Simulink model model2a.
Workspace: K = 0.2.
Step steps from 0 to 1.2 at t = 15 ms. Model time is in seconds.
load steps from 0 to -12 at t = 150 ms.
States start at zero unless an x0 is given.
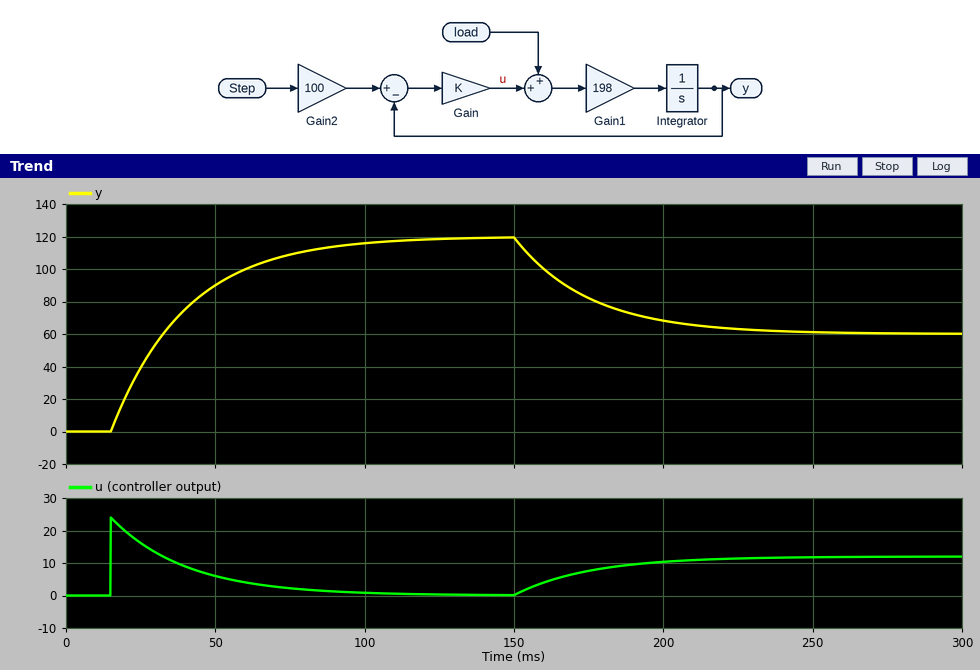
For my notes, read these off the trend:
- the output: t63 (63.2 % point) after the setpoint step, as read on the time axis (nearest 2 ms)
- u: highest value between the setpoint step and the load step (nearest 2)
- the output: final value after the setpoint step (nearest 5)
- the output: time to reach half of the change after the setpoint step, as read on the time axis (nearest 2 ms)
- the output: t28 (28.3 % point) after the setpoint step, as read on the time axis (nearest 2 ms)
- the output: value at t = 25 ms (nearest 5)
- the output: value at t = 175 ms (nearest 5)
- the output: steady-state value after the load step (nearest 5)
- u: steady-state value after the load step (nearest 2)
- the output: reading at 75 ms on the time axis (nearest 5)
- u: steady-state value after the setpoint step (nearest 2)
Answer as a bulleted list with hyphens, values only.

- 40 ms
- 24
- 120
- 32 ms
- 24 ms
- 40
- 80
- 60
- 12
- 110
- 0
